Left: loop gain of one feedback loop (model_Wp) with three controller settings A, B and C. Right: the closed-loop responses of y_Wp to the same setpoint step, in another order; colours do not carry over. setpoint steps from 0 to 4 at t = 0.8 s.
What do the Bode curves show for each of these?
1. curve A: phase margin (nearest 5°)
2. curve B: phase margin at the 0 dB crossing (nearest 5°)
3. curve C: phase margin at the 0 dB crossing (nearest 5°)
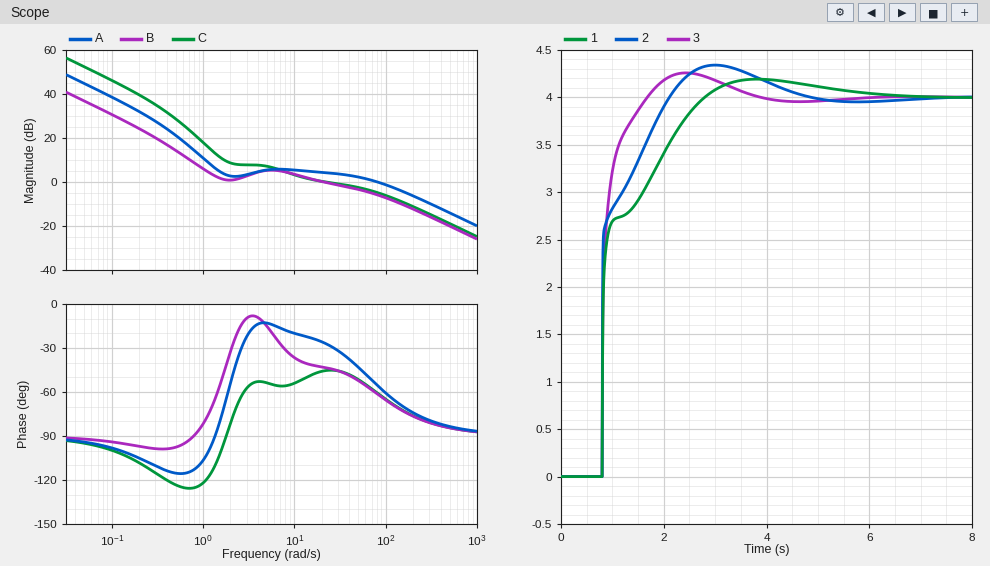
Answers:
125°
135°
135°
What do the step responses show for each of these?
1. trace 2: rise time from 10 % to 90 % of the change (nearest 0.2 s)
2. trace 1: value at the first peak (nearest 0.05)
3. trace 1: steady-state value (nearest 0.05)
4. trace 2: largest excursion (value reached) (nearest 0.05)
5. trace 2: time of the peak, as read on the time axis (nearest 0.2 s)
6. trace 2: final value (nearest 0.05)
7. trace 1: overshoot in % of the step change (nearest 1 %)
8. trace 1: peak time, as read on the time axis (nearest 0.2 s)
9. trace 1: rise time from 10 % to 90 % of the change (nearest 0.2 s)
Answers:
1.0 s
4.20
4.00
4.35
3.0 s
4.00
5 %
3.8 s
1.4 s
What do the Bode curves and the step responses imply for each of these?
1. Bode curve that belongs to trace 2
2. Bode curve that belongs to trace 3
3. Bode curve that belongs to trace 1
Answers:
A
C
B
